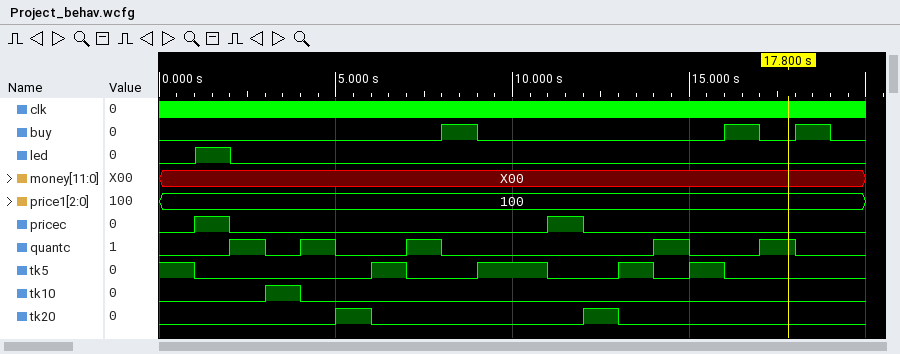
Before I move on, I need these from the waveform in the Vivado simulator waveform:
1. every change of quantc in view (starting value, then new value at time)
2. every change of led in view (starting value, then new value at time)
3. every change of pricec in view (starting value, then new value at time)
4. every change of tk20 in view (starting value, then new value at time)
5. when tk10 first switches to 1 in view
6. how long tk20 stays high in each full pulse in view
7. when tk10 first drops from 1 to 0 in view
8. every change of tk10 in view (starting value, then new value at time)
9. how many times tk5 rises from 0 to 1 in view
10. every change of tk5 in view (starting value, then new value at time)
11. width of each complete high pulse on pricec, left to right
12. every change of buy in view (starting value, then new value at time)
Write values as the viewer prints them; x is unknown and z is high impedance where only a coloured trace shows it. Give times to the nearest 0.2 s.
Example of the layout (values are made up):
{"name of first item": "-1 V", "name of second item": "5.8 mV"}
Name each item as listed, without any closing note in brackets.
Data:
{"every change of quantc in view": "0, 1 at 2 s, 0 at 3 s, 1 at 4 s, 0 at 5 s, 1 at 7 s, 0 at 8 s, 1 at 14 s, 0 at 15 s, 1 at 17 s, 0 at 18 s", "every change of led in view": "0, 1 at 1 s, 0 at 2 s", "every change of pricec in view": "0, 1 at 1 s, 0 at 2 s, 1 at 11 s, 0 at 12 s", "every change of tk20 in view": "0, 1 at 5 s, 0 at 6 s, 1 at 12 s, 0 at 13 s", "when tk10 first switches to 1 in view": "3 s", "how long tk20 stays high in each full pulse in view": "1 s, 1 s", "when tk10 first drops from 1 to 0 in view": "4 s", "every change of tk10 in view": "0, 1 at 3 s, 0 at 4 s", "how many times tk5 rises from 0 to 1 in view": "4", "every change of tk5 in view": "1, 0 at 1 s, 1 at 6 s, 0 at 7 s, 1 at 9 s, 0 at 11 s, 1 at 13 s, 0 at 14 s, 1 at 15 s, 0 at 16 s", "width of each complete high pulse on pricec, left to right": "1 s, 1 s", "every change of buy in view": "0, 1 at 8 s, 0 at 9 s, 1 at 16 s, 0 at 17 s, 1 at 18 s, 0 at 19 s"}
